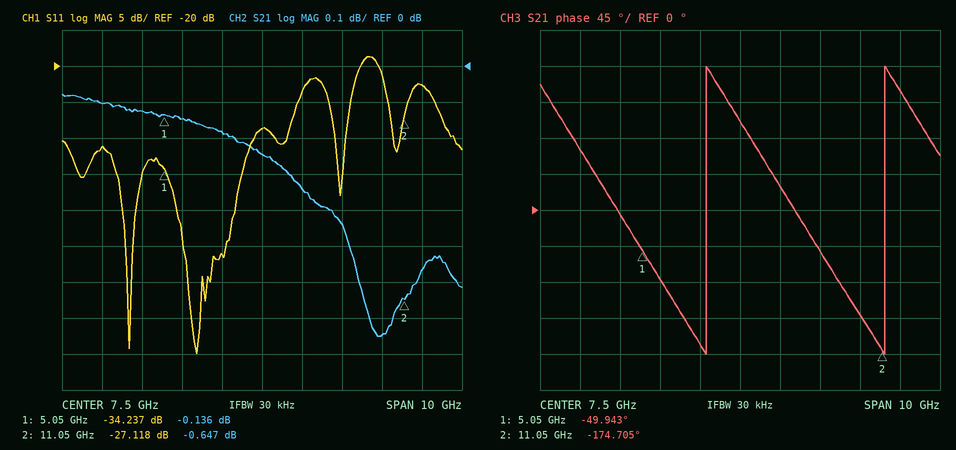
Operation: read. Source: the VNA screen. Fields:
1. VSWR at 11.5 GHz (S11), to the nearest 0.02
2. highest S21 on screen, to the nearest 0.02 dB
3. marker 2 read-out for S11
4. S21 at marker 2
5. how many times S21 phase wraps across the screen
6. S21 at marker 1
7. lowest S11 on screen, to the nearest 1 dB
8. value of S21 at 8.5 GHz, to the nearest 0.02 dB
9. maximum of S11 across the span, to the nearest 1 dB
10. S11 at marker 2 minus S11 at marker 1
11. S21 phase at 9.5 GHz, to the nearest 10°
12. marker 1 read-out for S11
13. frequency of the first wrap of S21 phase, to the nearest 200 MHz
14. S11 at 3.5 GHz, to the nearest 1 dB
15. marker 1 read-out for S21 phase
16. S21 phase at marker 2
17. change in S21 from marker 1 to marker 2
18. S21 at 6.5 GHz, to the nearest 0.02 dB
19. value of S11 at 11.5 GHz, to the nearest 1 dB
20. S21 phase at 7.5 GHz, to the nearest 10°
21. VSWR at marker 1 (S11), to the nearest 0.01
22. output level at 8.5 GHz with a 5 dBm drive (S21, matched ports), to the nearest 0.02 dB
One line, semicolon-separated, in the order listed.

1.16; -0.08 dB; -27.118 dB; -0.647 dB; 2; -0.136 dB; -60 dB; -0.34 dB; -19 dB; 7.119 dB; -50°; -34.237 dB; 6.6 GHz; -31 dB; -49.943°; -174.705°; -0.511 dB; -0.18 dB; -23 dB; 110°; 1.04; 4.66 dBm
